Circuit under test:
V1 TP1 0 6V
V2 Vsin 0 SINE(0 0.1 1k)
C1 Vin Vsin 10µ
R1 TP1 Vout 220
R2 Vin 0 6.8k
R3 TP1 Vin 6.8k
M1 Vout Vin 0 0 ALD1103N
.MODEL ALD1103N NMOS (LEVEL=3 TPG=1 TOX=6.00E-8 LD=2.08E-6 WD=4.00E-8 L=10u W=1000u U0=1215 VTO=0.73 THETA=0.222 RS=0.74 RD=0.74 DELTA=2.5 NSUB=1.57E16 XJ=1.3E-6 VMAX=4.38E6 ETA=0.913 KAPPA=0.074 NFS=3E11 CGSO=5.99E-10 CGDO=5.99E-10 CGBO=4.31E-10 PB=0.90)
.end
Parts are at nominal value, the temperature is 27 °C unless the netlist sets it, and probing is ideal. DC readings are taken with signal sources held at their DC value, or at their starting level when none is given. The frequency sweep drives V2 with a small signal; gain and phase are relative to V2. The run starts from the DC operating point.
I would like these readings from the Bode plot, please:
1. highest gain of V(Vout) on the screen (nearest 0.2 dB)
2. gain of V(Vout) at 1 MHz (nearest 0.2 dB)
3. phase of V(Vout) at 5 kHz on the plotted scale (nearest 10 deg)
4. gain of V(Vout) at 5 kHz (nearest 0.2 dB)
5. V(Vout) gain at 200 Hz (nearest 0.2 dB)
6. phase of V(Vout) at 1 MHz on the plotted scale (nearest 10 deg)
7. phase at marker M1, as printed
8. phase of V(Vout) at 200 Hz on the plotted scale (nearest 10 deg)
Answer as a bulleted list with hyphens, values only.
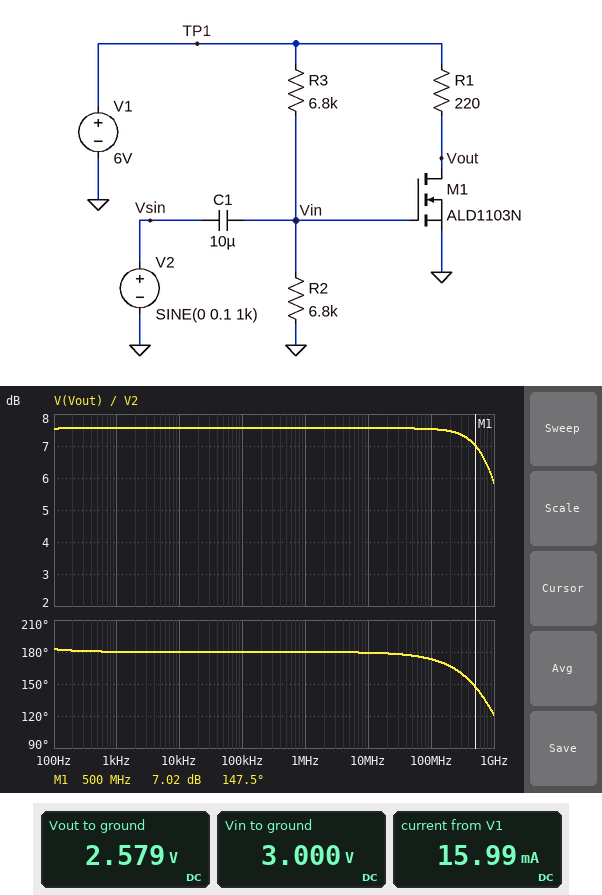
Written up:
- 7.6 dB
- 7.6 dB
- 180 deg
- 7.6 dB
- 7.6 dB
- 180 deg
- 147.5 deg
- 180 deg
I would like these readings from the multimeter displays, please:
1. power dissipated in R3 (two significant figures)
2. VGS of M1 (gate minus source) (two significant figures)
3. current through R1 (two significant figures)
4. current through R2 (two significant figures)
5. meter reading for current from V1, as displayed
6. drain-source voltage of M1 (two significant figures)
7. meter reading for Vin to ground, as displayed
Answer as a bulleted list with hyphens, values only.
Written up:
- 1.3 mW
- 3.0 V
- 16 mA
- 440 µA
- 15.99 mA
- 2.6 V
- 3.000 V
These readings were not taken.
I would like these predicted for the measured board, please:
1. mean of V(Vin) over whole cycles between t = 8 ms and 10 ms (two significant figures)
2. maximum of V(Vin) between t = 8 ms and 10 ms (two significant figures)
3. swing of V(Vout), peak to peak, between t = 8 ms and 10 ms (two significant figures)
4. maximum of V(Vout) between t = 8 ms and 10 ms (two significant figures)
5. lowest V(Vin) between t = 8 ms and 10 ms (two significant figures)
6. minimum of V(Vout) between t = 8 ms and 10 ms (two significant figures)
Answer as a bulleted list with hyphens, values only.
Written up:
- 3.0 V
- 3.1 V
- 480 mV
- 2.8 V
- 2.9 V
- 2.3 V
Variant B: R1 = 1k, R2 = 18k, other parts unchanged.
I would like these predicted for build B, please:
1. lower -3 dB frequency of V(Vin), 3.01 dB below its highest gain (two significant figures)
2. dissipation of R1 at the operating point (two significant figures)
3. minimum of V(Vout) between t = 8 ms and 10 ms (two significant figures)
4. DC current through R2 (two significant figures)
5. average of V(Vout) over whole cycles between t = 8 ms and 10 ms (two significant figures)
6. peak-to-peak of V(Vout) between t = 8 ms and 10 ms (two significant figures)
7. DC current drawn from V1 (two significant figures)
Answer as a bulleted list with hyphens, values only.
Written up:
- 3.2 Hz
- 33 mW
- 250 mV
- 240 µA
- 260 mV
- 8.2 mV
- 6.0 mA
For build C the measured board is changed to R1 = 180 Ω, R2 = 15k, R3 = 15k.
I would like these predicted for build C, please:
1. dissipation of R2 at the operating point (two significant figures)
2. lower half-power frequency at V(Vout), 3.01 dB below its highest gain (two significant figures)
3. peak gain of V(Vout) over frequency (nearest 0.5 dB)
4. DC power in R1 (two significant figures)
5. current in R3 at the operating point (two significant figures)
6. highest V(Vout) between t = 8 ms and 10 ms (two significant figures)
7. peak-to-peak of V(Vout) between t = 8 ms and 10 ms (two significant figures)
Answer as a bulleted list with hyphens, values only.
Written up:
- 600 µW
- 2.1 Hz
- 6.0 dB
- 44 mW
- 200 µA
- 3.4 V
- 390 mV
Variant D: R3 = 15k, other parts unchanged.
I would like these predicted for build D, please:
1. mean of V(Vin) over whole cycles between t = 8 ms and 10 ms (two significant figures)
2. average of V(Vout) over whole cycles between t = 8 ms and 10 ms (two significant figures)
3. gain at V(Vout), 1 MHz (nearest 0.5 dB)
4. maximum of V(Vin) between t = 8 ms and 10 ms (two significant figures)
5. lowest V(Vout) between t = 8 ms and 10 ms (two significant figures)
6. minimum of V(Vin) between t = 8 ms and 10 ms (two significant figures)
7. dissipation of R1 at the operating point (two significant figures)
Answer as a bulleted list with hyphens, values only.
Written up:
- 1.9 V
- 4.9 V
- 4.0 dB
- 2.0 V
- 4.7 V
- 1.8 V
- 5.7 mW
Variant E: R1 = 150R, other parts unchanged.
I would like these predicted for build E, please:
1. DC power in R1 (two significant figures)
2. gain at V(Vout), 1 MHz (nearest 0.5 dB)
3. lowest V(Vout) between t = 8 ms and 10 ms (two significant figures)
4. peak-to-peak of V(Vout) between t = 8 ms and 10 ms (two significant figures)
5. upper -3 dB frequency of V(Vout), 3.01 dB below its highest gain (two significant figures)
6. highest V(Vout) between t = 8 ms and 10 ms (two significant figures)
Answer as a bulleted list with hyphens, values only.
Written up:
- 37 mW
- 4.5 dB
- 3.5 V
- 330 mV
- 4.2 GHz
- 3.8 V
